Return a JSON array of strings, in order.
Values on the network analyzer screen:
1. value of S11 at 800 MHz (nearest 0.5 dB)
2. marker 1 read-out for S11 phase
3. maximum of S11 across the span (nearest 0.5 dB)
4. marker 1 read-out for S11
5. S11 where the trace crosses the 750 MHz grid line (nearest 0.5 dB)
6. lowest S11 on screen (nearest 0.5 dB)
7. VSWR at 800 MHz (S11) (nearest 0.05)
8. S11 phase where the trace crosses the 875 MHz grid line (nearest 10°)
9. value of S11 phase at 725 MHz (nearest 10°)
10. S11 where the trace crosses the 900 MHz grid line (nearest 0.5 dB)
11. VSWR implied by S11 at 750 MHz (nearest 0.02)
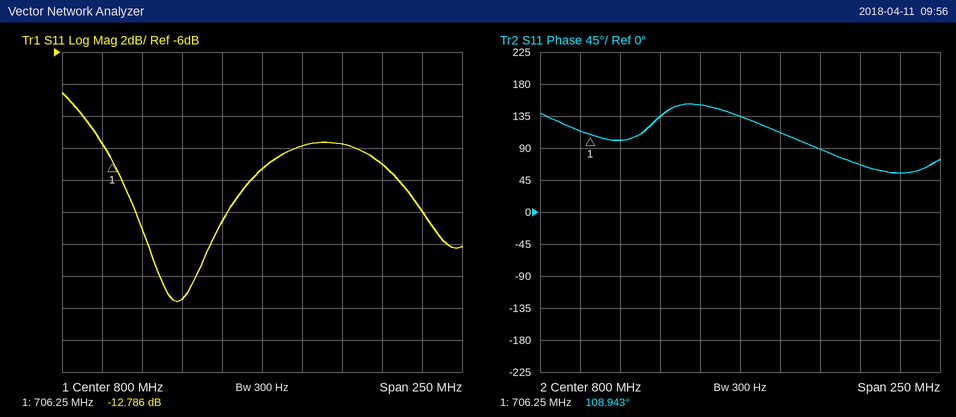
["-13.5 dB", "108.943°", "-8.5 dB", "-12.786 dB", "-21.5 dB", "-21.5 dB", "1.55", "70°", "100°", "-16.0 dB", "1.18"]
